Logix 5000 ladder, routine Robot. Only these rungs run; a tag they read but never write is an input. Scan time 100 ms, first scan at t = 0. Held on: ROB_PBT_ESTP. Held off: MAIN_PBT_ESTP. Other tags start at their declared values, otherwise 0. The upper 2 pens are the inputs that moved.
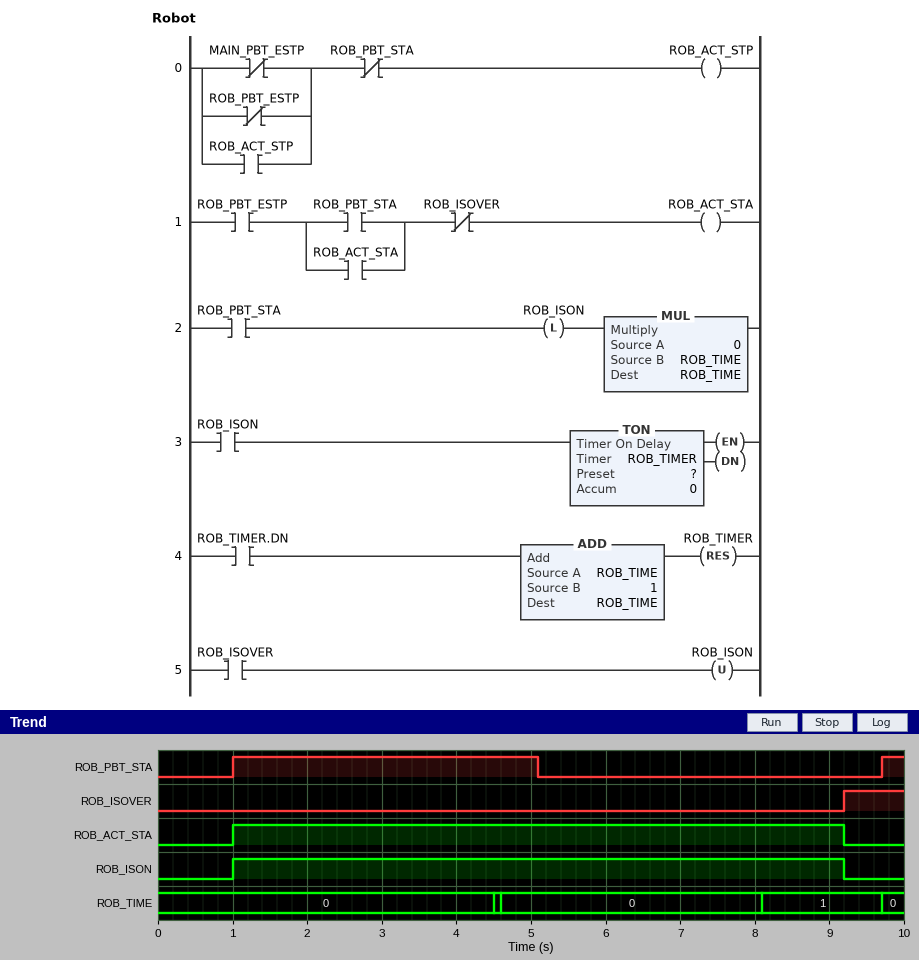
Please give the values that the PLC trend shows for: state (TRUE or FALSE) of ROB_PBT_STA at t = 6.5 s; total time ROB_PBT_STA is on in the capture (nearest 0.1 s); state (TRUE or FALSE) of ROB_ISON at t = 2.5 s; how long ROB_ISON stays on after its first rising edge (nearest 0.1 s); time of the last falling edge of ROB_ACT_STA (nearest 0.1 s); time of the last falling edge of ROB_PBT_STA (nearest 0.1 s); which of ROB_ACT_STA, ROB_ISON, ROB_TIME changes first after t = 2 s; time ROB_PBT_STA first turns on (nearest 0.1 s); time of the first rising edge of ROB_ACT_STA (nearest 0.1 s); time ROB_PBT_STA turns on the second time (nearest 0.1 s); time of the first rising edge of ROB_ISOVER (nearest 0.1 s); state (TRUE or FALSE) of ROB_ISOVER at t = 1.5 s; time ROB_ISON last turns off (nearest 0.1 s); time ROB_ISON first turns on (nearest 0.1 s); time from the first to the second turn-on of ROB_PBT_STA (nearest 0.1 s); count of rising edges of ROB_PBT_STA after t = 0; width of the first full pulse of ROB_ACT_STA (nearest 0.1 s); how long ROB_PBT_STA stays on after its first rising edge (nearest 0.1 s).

FALSE
4.4 s
TRUE
8.2 s
9.2 s
5.1 s
ROB_TIME
1.0 s
1.0 s
9.7 s
9.2 s
FALSE
9.2 s
1.0 s
8.7 s
2
8.2 s
4.1 s
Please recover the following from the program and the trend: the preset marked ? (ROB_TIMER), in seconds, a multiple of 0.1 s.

3.5 s
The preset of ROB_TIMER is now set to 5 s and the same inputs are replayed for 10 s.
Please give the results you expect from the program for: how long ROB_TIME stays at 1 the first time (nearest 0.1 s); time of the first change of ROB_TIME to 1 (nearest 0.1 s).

3.7 s
6.0 s
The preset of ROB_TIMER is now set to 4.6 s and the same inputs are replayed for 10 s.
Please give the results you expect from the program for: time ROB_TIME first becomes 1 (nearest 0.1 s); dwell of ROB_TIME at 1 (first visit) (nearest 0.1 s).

5.6 s
4.1 s
